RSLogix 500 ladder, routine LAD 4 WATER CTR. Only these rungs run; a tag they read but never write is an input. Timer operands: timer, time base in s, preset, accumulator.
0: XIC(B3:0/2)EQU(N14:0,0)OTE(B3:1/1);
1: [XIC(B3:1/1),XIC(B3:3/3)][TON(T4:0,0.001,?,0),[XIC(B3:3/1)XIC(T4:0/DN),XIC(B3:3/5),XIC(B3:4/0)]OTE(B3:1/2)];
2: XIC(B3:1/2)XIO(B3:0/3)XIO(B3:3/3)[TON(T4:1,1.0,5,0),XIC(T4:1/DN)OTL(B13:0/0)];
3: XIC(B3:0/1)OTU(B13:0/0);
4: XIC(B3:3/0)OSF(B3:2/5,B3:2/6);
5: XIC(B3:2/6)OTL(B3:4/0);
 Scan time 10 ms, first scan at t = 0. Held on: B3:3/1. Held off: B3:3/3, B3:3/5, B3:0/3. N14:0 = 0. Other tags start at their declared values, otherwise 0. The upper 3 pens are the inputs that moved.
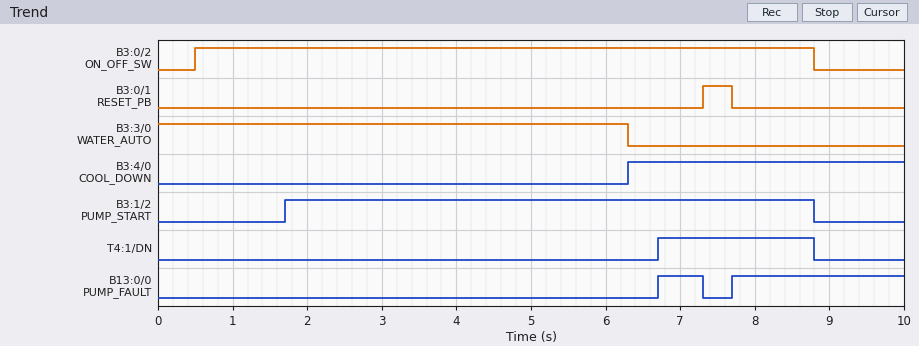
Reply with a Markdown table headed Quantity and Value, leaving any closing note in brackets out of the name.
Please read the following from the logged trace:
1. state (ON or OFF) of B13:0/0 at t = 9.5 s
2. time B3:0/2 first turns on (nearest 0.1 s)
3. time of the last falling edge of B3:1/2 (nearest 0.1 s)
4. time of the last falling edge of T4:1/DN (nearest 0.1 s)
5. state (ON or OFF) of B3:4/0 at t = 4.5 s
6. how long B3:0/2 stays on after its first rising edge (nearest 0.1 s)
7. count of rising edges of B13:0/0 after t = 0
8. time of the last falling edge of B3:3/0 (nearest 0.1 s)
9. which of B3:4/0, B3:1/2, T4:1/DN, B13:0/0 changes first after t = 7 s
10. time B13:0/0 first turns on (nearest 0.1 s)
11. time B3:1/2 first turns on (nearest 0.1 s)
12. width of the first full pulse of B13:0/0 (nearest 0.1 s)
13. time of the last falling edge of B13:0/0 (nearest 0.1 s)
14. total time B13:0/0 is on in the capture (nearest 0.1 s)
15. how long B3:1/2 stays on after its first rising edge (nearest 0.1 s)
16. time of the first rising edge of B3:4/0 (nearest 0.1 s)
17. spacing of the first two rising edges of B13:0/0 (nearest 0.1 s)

| Quantity | Value |
|---|---|
| state (ON or OFF) of B13:0/0 at t = 9.5 s | ON |
| time B3:0/2 first turns on | 0.5 s |
| time of the last falling edge of B3:1/2 | 8.8 s |
| time of the last falling edge of T4:1/DN | 8.8 s |
| state (ON or OFF) of B3:4/0 at t = 4.5 s | OFF |
| how long B3:0/2 stays on after its first rising edge | 8.3 s |
| count of rising edges of B13:0/0 after t = 0 | 2 |
| time of the last falling edge of B3:3/0 | 6.3 s |
| which of B3:4/0, B3:1/2, T4:1/DN, B13:0/0 changes first after t = 7 s | B13:0/0 |
| time B13:0/0 first turns on | 6.7 s |
| time B3:1/2 first turns on | 1.7 s |
| width of the first full pulse of B13:0/0 | 0.6 s |
| time of the last falling edge of B13:0/0 | 7.3 s |
| total time B13:0/0 is on in the capture | 2.9 s |
| how long B3:1/2 stays on after its first rising edge | 7.1 s |
| time of the first rising edge of B3:4/0 | 6.3 s |
| spacing of the first two rising edges of B13:0/0 | 1.0 s |
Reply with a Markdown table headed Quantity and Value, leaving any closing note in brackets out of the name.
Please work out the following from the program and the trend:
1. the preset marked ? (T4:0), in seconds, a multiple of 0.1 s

| Quantity | Value |
|---|---|
| the preset marked ? (T4:0), in seconds, a multiple of 0.1 s | 1.2 s |
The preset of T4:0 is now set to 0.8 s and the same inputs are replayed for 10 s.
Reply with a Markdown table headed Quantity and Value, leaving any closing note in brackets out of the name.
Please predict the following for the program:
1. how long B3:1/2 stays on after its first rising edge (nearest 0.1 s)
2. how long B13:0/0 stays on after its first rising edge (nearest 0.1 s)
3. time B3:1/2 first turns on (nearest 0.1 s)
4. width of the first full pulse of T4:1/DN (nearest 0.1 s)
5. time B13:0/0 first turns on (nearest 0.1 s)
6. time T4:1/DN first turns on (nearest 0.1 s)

| Quantity | Value |
|---|---|
| how long B3:1/2 stays on after its first rising edge | 7.5 s |
| how long B13:0/0 stays on after its first rising edge | 1.0 s |
| time B3:1/2 first turns on | 1.3 s |
| width of the first full pulse of T4:1/DN | 2.5 s |
| time B13:0/0 first turns on | 6.3 s |
| time T4:1/DN first turns on | 6.3 s |
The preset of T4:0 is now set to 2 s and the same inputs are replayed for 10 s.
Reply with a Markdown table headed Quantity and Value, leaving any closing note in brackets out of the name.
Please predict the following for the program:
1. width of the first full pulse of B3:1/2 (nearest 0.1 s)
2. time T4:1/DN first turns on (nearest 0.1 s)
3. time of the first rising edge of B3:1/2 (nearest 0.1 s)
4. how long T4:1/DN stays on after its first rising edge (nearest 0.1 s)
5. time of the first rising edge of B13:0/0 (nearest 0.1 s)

| Quantity | Value |
|---|---|
| width of the first full pulse of B3:1/2 | 6.3 s |
| time T4:1/DN first turns on | 7.5 s |
| time of the first rising edge of B3:1/2 | 2.5 s |
| how long T4:1/DN stays on after its first rising edge | 1.3 s |
| time of the first rising edge of B13:0/0 | 7.7 s |
